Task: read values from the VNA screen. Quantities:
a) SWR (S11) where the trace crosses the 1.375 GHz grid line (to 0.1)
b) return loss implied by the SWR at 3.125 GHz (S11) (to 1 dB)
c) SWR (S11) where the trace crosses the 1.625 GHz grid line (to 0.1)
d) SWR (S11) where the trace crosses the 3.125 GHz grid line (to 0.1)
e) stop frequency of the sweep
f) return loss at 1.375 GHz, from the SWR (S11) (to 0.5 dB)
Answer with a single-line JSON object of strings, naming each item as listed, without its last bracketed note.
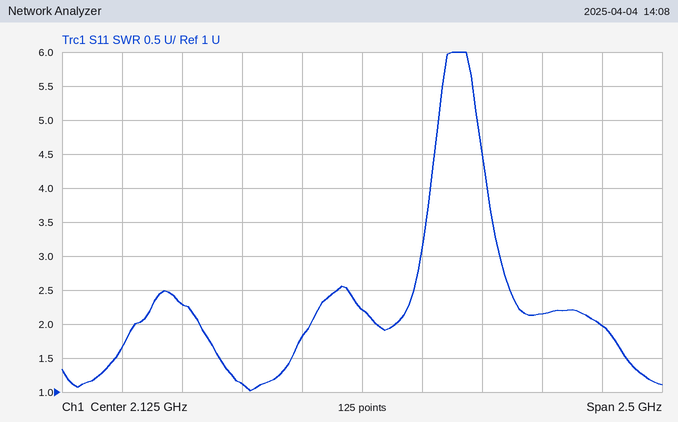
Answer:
{"SWR (S11) where the trace crosses the 1.375 GHz grid line": "2.3", "return loss implied by the SWR at 3.125 GHz (S11)": "10 dB", "SWR (S11) where the trace crosses the 1.625 GHz grid line": "1.1", "SWR (S11) where the trace crosses the 3.125 GHz grid line": "2.0", "stop frequency of the sweep": "3.375 GHz", "return loss at 1.375 GHz, from the SWR (S11)": "8.0 dB"}
